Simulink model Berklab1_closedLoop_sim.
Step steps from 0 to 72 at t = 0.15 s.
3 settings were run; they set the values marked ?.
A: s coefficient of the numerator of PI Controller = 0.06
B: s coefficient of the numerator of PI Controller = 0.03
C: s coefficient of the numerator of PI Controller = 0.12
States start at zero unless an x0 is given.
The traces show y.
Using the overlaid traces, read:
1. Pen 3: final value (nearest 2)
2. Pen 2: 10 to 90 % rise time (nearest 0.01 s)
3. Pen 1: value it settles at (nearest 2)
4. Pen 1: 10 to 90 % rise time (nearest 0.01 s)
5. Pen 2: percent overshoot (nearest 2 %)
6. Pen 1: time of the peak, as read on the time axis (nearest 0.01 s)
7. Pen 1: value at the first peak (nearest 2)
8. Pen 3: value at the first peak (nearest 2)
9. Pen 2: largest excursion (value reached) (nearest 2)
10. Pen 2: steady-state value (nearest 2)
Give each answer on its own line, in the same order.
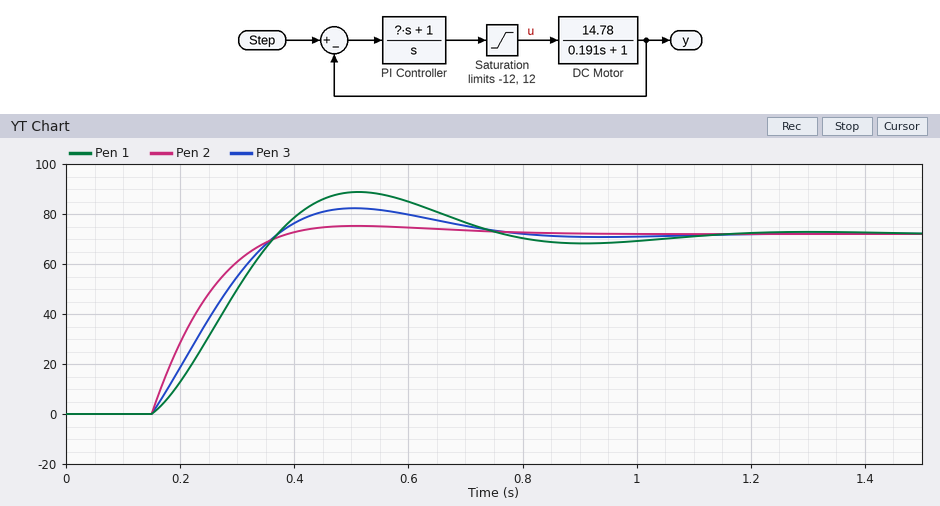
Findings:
72
0.16 s
72
0.16 s
4 %
0.51 s
88
82
76
72
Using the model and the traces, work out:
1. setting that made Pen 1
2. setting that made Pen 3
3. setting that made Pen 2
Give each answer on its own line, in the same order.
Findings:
B
A
C
